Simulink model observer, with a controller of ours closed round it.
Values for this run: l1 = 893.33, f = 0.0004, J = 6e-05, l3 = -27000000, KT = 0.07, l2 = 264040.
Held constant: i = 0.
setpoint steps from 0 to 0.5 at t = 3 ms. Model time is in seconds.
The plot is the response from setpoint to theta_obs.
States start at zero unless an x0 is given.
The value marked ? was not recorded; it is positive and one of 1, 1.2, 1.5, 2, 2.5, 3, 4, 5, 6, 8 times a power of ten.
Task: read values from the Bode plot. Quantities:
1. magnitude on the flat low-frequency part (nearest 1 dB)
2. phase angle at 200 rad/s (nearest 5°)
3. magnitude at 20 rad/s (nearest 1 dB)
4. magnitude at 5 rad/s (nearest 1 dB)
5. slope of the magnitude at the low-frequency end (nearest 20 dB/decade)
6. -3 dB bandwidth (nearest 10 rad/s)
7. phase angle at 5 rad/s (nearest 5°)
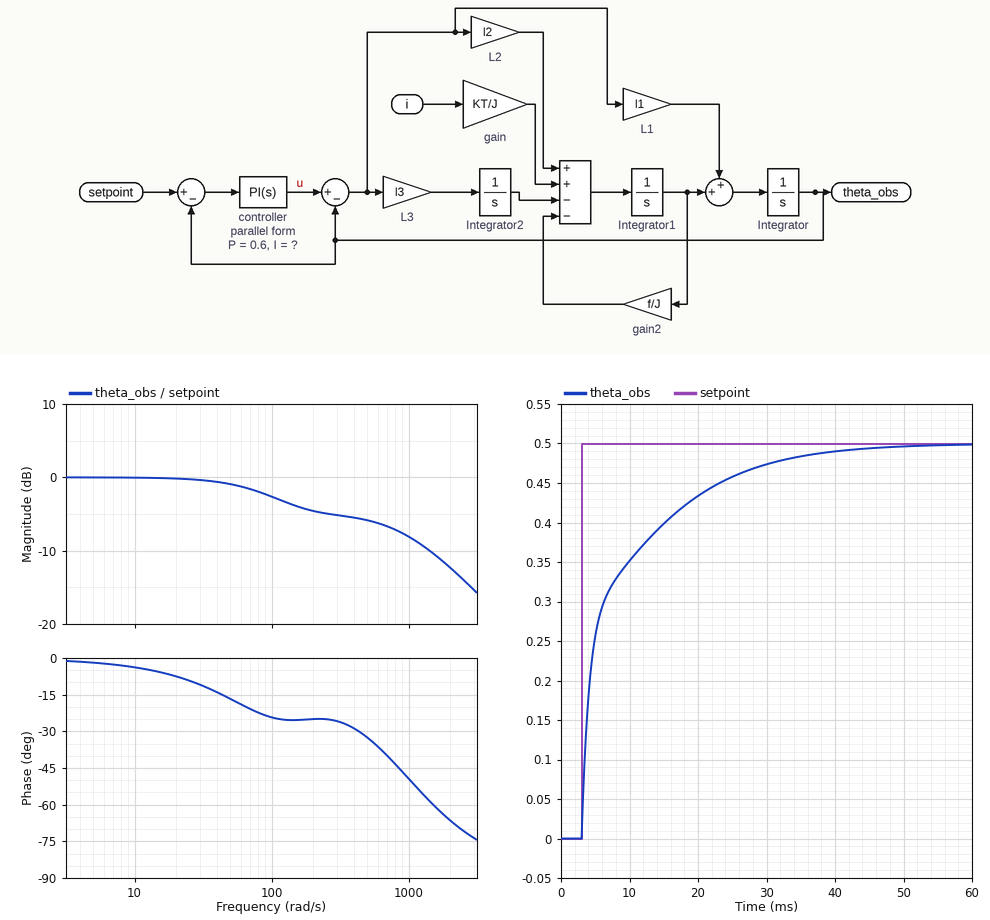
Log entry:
0 dB
-25°
0 dB
0 dB
0 dB/decade
110 rad/s
0°
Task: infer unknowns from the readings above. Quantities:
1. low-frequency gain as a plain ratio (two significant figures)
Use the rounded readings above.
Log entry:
1.0
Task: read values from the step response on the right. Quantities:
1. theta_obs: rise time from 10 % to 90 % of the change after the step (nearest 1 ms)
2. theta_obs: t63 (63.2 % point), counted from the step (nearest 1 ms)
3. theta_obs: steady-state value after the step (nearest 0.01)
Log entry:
20 ms
4 ms
0.50
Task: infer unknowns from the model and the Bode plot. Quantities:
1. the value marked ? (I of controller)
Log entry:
150
